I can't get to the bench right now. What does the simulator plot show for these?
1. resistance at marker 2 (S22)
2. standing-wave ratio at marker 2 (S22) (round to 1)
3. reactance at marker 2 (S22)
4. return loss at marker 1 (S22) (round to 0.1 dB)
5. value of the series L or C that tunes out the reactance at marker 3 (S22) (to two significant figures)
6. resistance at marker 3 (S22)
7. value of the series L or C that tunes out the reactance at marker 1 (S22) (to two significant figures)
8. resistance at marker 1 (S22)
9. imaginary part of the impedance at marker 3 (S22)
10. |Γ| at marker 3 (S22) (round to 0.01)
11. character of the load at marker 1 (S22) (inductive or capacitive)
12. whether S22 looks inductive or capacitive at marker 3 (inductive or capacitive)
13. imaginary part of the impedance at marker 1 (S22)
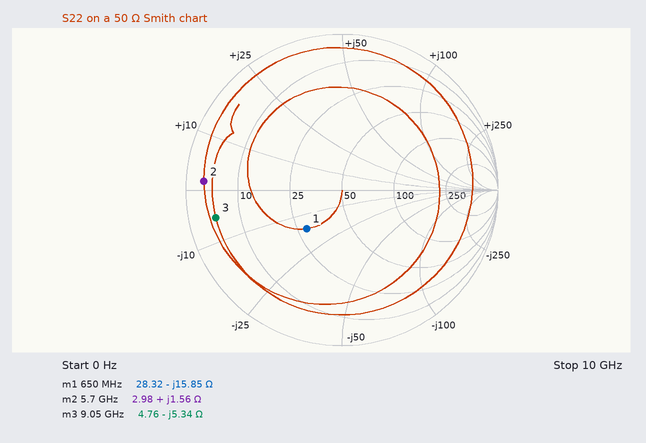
2.98 Ω
17
+1.56 Ω
9.5 dB
94 pH
4.76 Ω
3.9 nH
28.32 Ω
-5.34 Ω
0.83
capacitive
capacitive
-15.85 Ω
